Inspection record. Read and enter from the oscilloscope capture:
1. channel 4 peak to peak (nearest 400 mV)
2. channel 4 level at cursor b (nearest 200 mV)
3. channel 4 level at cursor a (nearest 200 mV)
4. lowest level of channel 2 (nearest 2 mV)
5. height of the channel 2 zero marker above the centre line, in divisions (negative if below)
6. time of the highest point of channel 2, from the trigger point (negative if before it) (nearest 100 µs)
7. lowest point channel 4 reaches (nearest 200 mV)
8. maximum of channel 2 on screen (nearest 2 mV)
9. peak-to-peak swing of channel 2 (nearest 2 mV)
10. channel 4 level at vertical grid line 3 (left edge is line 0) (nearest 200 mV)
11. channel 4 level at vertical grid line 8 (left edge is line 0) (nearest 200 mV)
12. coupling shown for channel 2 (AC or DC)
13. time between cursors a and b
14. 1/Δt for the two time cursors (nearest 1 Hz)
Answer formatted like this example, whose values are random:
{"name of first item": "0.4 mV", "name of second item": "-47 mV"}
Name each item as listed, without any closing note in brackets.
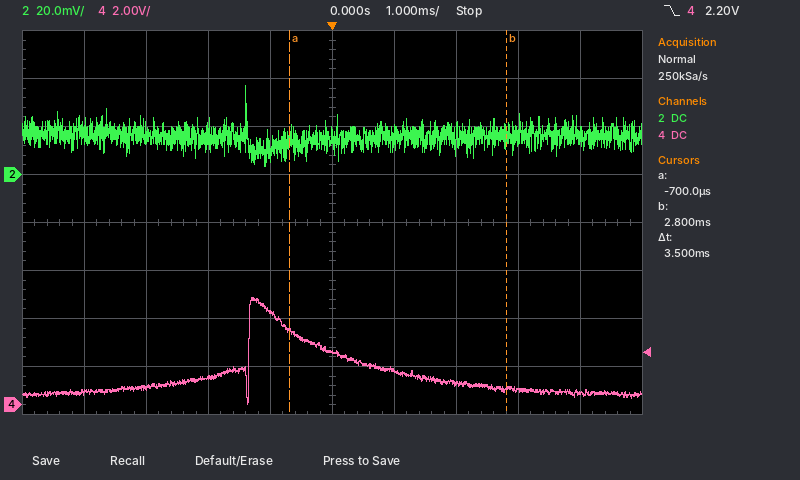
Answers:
{"channel 4 peak to peak": "4.4 V", "channel 4 level at cursor b": "600 mV", "channel 4 level at cursor a": "3.0 V", "lowest level of channel 2": "4 mV", "height of the channel 2 zero marker above the centre line, in divisions": "+1.0 div", "time of the highest point of channel 2, from the trigger point (negative if before it)": "-1.4 ms", "lowest point channel 4 reaches": "0.0 V", "maximum of channel 2 on screen": "38 mV", "peak-to-peak swing of channel 2": "34 mV", "channel 4 level at vertical grid line 3 (left edge is line 0)": "1.2 V", "channel 4 level at vertical grid line 8 (left edge is line 0)": "600 mV", "coupling shown for channel 2": "DC", "time between cursors a and b": "3.5 ms", "1/Δt for the two time cursors": "286 Hz"}
